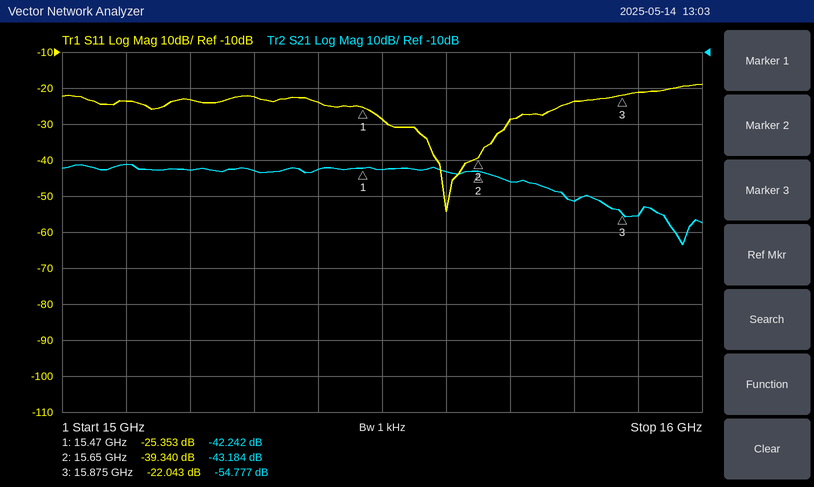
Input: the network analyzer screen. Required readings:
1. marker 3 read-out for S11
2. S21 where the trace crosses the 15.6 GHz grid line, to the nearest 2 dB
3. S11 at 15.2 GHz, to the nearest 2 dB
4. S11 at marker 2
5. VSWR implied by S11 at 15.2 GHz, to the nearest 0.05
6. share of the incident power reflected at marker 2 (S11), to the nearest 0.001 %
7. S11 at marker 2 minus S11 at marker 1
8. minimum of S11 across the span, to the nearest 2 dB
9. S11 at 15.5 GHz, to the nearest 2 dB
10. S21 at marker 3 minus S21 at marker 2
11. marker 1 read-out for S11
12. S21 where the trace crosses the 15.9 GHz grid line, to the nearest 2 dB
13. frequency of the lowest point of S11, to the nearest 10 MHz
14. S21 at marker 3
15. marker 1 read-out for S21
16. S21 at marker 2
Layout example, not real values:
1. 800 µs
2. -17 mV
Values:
1. -22.043 dB
2. -44 dB
3. -24 dB
4. -39.340 dB
5. 1.15
6. 0.012 %
7. -13.987 dB
8. -54 dB
9. -28 dB
10. -11.593 dB
11. -25.353 dB
12. -56 dB
13. 15.60 GHz
14. -54.777 dB
15. -42.242 dB
16. -43.184 dB
